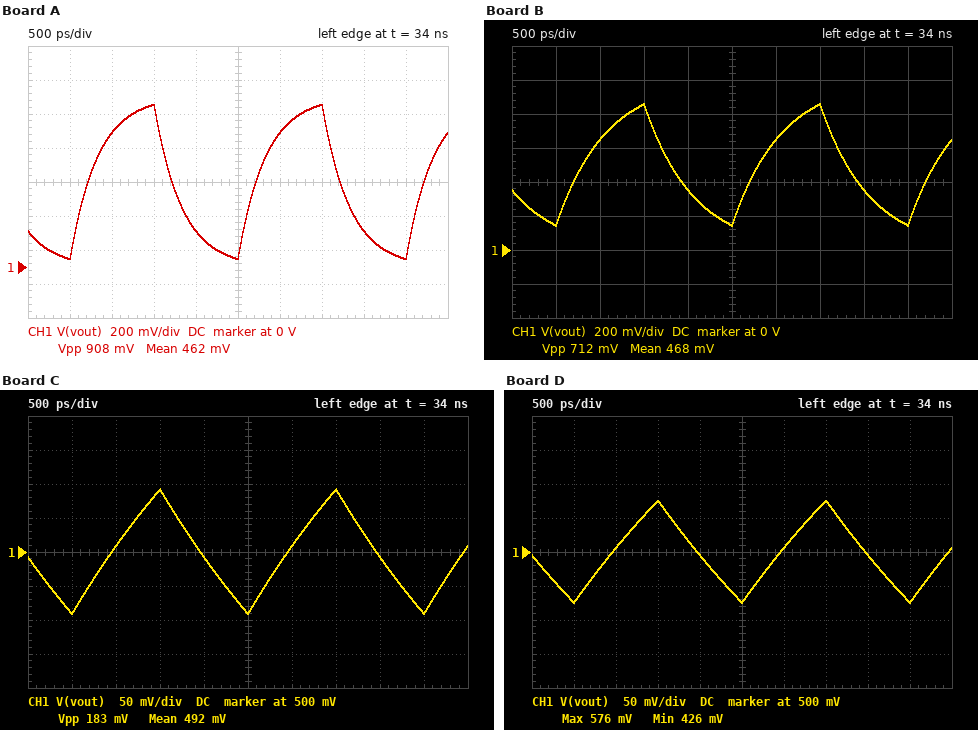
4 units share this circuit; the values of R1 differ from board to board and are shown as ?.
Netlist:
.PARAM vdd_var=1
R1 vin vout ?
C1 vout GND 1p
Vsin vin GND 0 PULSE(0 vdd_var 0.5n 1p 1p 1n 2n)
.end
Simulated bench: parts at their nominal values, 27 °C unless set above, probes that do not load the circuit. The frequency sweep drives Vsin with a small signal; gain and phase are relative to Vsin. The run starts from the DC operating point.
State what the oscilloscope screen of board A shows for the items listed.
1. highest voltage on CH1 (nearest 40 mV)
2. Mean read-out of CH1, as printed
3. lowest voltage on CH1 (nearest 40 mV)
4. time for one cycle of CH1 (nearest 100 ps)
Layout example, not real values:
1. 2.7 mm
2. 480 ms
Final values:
1. 960 mV
2. 462 mV
3. 40 mV
4. 2.0 ns
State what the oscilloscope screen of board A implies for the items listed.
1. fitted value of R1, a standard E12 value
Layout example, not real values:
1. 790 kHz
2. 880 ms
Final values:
1. 330 Ω
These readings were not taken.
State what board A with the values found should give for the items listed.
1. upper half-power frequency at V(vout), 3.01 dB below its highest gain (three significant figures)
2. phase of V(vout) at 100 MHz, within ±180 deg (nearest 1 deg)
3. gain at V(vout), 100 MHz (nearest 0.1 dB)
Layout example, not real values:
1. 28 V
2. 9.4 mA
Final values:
1. 482 MHz
2. -12 deg
3. -0.2 dB
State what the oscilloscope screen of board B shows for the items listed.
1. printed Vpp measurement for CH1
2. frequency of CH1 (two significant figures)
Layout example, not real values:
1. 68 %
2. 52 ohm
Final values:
1. 712 mV
2. 500 MHz
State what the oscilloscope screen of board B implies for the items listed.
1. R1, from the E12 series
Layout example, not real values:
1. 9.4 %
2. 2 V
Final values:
1. 560 Ω
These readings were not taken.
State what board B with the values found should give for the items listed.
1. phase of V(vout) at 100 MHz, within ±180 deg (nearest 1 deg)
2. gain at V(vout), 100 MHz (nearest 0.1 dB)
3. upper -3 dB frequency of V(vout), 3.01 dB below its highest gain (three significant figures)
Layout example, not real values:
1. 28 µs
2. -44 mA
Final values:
1. -19 deg
2. -0.5 dB
3. 284 MHz
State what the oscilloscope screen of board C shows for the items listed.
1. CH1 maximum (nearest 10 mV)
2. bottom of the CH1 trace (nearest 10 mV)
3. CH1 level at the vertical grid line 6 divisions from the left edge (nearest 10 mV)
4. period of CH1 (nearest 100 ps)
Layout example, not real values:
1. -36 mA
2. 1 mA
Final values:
1. 590 mV
2. 410 mV
3. 510 mV
4. 2.0 ns
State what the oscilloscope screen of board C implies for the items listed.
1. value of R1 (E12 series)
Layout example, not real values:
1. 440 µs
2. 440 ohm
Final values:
1. 2.7 kΩ
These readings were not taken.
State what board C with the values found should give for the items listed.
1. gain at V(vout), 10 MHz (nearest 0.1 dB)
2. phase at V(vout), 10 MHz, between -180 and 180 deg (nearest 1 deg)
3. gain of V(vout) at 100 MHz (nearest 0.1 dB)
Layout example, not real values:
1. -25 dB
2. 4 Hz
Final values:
1. -0.1 dB
2. -10 deg
3. -5.9 dB
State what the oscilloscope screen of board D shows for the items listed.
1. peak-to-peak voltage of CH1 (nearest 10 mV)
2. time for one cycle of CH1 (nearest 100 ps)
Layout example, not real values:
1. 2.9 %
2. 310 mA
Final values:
1. 150 mV
2. 2.0 ns
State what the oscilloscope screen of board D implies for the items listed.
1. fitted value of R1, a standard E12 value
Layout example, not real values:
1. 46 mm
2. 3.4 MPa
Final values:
1. 3.3 kΩ
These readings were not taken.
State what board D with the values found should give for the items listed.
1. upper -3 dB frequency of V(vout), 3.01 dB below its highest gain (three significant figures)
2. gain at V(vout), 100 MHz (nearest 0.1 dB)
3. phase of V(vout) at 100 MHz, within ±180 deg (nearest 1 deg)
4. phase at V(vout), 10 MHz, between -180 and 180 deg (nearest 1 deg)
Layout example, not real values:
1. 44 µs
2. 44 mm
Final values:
1. 48.2 MHz
2. -7.2 dB
3. -64 deg
4. -12 deg
